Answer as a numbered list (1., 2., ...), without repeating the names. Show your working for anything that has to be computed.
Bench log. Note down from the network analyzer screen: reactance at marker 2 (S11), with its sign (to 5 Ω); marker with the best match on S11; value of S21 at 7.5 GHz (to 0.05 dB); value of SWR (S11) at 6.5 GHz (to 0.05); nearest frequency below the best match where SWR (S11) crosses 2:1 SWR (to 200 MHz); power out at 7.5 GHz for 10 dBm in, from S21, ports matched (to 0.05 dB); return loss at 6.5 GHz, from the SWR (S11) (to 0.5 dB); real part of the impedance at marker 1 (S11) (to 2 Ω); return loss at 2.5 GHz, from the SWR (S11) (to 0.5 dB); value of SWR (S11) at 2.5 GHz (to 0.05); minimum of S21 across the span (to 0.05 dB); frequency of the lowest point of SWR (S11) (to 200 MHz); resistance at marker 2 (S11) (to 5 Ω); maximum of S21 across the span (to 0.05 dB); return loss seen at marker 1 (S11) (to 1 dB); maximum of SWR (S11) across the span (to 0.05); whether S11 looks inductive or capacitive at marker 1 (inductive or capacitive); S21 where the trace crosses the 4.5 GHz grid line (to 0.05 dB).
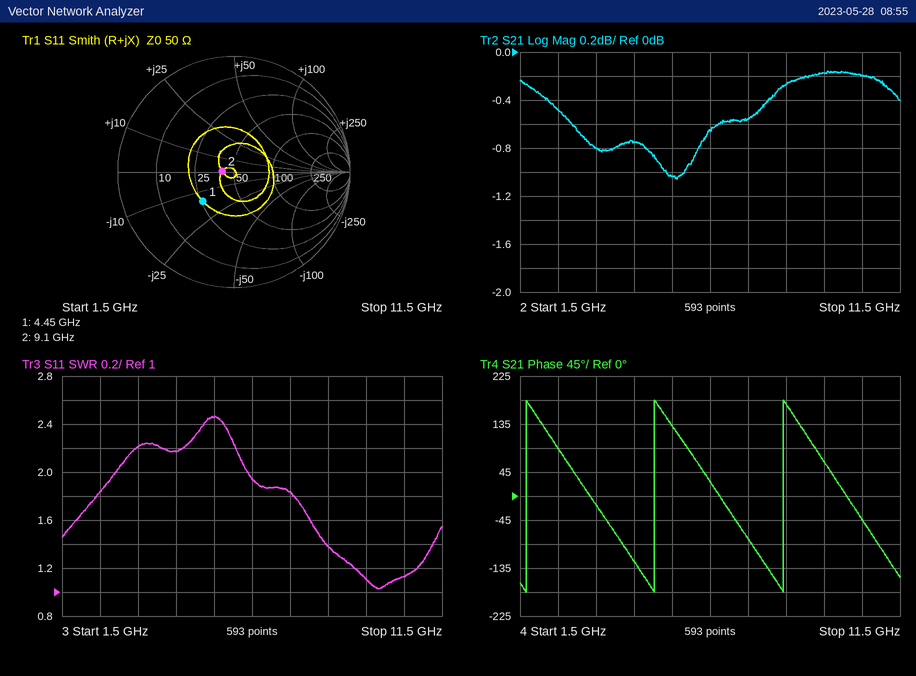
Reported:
1. 0 Ω
2. marker 2
3. -0.55 dB
4. 1.95
5. 6.4 GHz
6. 10 dBm + (-0.55 dB) = 9.45 dBm
7. −20 log10((1.95 − 1)/(1.95 + 1)) ≈ 9.84 dB, so 10.0 dB to the nearest 0.5 dB
8. 26 Ω
9. −20 log10((1.85 − 1)/(1.85 + 1)) ≈ 10.5 dB
10. 1.85
11. -1.05 dB
12. 9.8 GHz
13. 40 Ω
14. -0.15 dB
15. 9 dB
16. 2.45
17. capacitive
18. -0.75 dB
